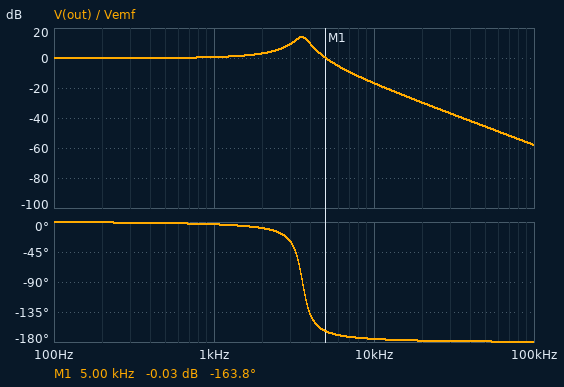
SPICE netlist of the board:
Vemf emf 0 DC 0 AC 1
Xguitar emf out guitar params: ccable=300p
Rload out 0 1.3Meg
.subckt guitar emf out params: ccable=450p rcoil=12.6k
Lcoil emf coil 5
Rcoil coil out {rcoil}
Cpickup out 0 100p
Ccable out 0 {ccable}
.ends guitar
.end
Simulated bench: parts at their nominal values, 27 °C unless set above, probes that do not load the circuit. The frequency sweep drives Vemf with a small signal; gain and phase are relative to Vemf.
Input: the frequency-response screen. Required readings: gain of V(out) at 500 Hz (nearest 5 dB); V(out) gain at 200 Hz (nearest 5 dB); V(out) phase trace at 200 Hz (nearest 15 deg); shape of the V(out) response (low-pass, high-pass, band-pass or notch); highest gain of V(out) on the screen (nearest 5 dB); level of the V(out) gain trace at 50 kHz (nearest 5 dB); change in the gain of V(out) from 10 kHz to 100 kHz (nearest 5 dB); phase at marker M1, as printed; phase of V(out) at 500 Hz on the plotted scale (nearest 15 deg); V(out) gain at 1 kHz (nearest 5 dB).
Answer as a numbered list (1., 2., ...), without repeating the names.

1. 0 dB
2. 0 dB
3. 0 deg
4. low-pass
5. 15 dB
6. -45 dB
7. -40 dB
8. -163.8 deg
9. 0 deg
10. 0 dB
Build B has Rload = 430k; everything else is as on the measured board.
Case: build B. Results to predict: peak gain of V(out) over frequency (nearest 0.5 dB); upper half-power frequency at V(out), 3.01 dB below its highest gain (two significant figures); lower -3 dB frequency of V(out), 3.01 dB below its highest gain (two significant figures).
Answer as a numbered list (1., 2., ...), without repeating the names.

1. 8.5 dB
2. 4.1 kHz
3. 2.7 kHz
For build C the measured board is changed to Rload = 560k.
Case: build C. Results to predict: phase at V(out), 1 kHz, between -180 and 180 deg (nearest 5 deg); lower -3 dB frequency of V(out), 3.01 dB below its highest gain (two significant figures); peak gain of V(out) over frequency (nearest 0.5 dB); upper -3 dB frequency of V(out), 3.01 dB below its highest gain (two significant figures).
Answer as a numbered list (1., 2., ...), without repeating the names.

1. -5 deg
2. 2.9 kHz
3. 10.0 dB
4. 4.0 kHz
